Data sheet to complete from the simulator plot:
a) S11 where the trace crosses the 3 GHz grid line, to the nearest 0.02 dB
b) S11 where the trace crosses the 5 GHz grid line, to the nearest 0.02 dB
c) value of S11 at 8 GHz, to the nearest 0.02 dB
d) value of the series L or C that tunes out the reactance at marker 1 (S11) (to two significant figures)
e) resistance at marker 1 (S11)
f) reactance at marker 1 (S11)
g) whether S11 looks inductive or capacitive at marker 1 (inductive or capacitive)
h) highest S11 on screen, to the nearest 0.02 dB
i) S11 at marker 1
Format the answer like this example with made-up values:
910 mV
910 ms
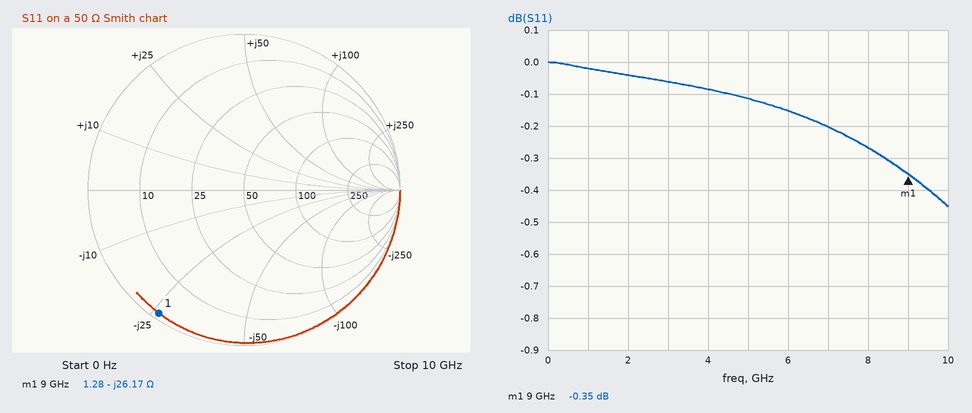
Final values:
-0.06 dB
-0.12 dB
-0.26 dB
460 pH
1.28 Ω
-26.17 Ω
capacitive
0.00 dB
-0.35 dB
